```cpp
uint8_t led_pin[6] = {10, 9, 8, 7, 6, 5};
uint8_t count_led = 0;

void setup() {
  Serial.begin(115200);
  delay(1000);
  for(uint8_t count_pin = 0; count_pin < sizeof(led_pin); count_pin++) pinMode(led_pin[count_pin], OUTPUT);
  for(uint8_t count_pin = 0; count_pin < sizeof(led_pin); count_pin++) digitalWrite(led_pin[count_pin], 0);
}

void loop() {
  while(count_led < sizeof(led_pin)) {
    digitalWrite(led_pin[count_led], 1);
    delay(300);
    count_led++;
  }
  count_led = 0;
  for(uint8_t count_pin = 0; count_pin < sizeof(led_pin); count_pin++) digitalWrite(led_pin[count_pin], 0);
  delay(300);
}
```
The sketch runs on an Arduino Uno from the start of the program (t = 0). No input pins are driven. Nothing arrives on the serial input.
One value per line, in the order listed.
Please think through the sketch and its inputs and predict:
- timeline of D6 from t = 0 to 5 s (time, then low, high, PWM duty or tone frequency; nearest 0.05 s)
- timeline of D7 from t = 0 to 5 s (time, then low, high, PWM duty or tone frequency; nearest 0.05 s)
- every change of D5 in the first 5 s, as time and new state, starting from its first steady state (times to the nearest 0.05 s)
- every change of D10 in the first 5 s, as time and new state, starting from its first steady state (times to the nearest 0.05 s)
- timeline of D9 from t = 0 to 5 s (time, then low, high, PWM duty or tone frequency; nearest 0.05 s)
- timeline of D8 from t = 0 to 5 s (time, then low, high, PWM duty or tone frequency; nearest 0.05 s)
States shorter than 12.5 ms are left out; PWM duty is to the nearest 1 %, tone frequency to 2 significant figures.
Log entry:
1 s low; 2.2 s high; 2.8 s low; 4.3 s high; 4.9 s low
1 s low; 1.9 s high; 2.8 s low; 4 s high; 4.9 s low
1 s low; 2.5 s high; 2.8 s low; 4.6 s high; 4.9 s low
1 s high; 2.8 s low; 3.1 s high; 4.9 s low
1 s low; 1.3 s high; 2.8 s low; 3.4 s high; 4.9 s low
1 s low; 1.6 s high; 2.8 s low; 3.7 s high; 4.9 s low
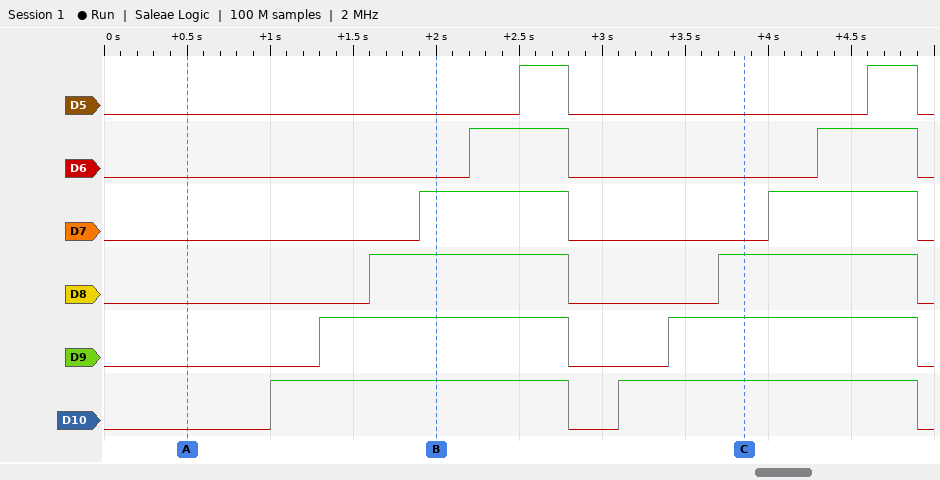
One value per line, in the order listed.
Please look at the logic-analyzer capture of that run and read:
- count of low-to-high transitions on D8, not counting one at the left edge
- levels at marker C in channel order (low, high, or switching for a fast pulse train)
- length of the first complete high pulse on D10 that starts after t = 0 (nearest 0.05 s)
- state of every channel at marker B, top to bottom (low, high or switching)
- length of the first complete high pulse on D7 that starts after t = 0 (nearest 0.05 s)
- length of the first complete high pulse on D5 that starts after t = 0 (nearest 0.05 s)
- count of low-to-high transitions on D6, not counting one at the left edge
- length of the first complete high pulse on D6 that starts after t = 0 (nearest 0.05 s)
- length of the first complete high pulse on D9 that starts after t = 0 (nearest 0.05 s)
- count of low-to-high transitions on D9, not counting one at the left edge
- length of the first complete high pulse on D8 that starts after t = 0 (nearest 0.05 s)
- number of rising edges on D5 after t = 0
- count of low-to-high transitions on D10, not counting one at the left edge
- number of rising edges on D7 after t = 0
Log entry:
2
D5 low, D6 low, D7 low, D8 high, D9 high, D10 high
1.80 s
D5 low, D6 low, D7 high, D8 high, D9 high, D10 high
0.90 s
0.30 s
2
0.60 s
1.50 s
2
1.20 s
2
2
2
